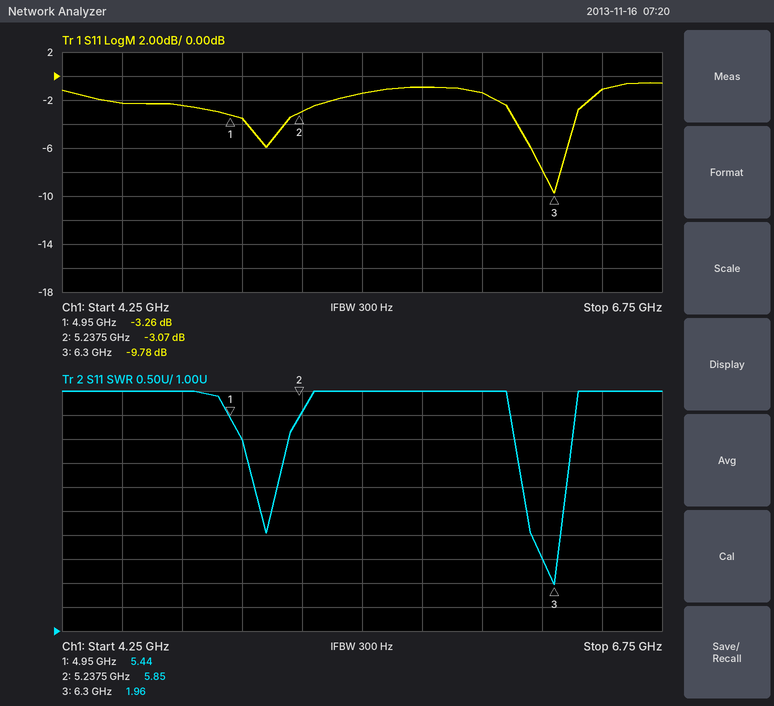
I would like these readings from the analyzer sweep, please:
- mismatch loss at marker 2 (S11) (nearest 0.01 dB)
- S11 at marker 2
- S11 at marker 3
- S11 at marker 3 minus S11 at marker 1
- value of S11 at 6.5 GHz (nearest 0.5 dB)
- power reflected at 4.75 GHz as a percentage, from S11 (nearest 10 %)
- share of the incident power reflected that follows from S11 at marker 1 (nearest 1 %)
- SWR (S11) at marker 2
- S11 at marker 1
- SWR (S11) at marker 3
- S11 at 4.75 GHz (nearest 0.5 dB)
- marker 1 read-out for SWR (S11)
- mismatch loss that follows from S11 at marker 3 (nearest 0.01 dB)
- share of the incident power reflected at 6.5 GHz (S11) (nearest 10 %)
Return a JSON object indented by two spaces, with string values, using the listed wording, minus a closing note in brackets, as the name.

{
  "mismatch loss at marker 2 (S11)": "2.95 dB",
  "S11 at marker 2": "-3.07 dB",
  "S11 at marker 3": "-9.78 dB",
  "S11 at marker 3 minus S11 at marker 1": "-6.52 dB",
  "value of S11 at 6.5 GHz": "-1.0 dB",
  "power reflected at 4.75 GHz as a percentage, from S11": "60 %",
  "share of the incident power reflected that follows from S11 at marker 1": "47 %",
  "SWR (S11) at marker 2": "5.85",
  "S11 at marker 1": "-3.26 dB",
  "SWR (S11) at marker 3": "1.96",
  "S11 at 4.75 GHz": "-2.5 dB",
  "marker 1 read-out for SWR": "5.44",
  "mismatch loss that follows from S11 at marker 3": "0.48 dB",
  "share of the incident power reflected at 6.5 GHz (S11)": "80 %"
}
